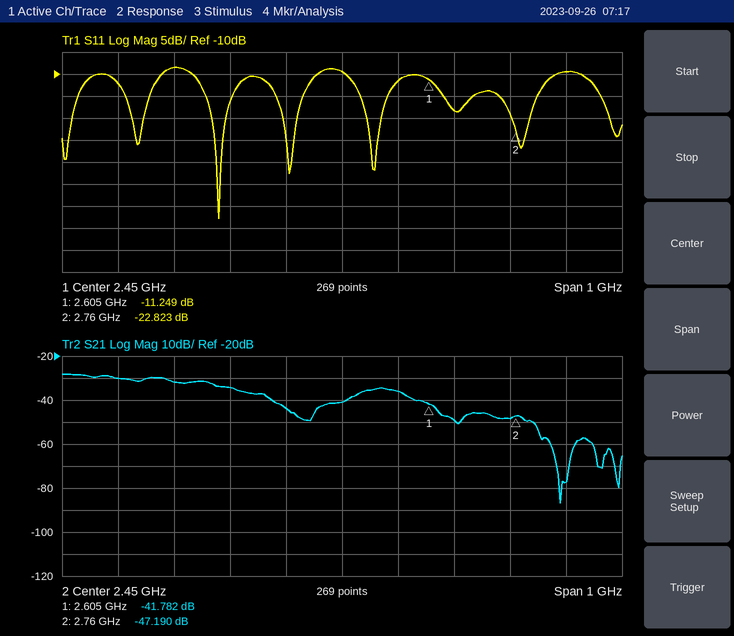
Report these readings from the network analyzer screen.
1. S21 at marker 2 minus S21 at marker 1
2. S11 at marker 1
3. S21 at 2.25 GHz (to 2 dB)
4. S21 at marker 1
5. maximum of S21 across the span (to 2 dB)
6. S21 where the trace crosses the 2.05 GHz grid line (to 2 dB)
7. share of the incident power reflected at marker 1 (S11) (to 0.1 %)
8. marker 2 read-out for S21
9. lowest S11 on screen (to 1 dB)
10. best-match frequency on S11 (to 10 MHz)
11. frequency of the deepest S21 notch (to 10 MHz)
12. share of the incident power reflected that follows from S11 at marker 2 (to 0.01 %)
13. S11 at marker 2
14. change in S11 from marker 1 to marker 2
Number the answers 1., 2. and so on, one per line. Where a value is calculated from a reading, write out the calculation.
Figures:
1. -47.19 − (-41.782) = -5.408 dB
2. -11.249 dB
3. -34 dB
4. -41.782 dB
5. -28 dB
6. -30 dB
7. 10^(-11.249/10) ≈ 7.5 %
8. -47.190 dB
9. -43 dB
10. 2.23 GHz
11. 2.84 GHz
12. 10^(-22.823/10) ≈ 0.52 %
13. -22.823 dB
14. -22.823 − (-11.249) = -11.574 dB
